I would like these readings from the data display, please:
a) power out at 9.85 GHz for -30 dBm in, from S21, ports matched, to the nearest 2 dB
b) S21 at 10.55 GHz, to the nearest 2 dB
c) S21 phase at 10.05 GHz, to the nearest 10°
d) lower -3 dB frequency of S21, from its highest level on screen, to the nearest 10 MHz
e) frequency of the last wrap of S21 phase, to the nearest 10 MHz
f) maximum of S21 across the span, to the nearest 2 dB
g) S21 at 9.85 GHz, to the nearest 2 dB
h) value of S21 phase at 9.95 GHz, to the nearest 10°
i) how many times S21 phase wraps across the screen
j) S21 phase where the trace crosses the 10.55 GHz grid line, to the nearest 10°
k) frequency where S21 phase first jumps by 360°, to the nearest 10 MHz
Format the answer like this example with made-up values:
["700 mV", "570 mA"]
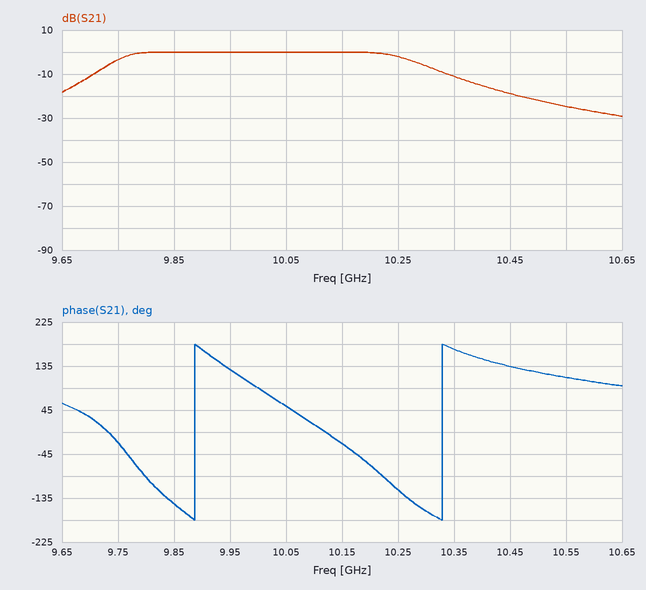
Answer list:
["-30 dBm", "-24 dB", "50°", "9.75 GHz", "10.33 GHz", "0 dB", "0 dB", "130°", "2", "110°", "9.89 GHz"]
